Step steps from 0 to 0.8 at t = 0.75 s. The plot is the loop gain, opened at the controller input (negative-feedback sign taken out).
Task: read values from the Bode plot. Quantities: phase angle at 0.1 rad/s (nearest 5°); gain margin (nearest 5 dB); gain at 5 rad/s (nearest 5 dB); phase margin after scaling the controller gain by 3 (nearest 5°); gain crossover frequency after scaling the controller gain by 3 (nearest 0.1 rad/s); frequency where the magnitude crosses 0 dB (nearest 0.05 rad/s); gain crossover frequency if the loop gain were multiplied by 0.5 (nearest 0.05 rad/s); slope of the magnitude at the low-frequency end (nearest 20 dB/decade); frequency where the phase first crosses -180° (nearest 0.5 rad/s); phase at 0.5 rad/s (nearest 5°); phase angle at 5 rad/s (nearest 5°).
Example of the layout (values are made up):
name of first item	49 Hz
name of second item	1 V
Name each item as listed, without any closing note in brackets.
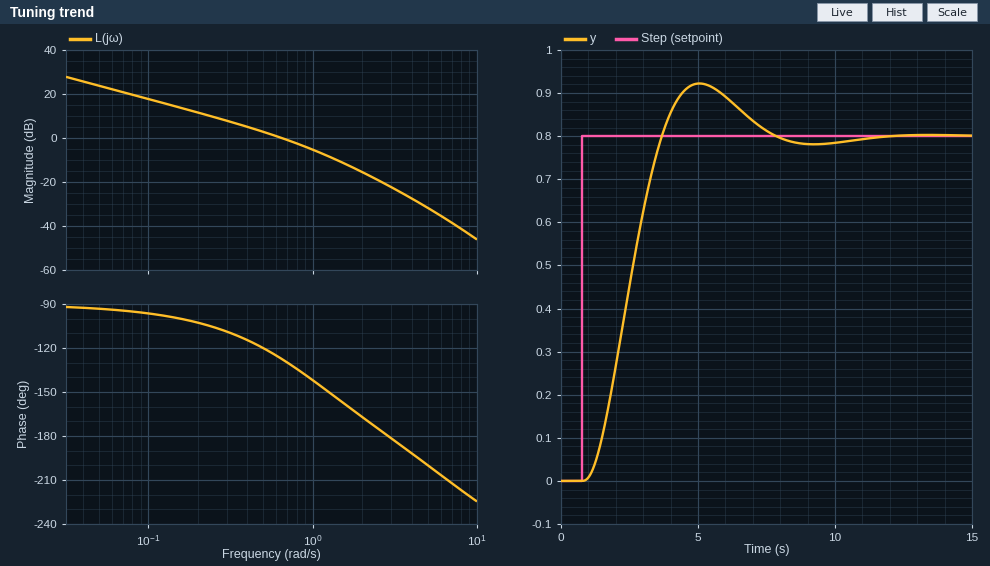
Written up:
phase angle at 0.1 rad/s	-95°
gain margin	20 dB
gain at 5 rad/s	-30 dB
phase margin after scaling the controller gain by 3	25°
gain crossover frequency after scaling the controller gain by 3	1.4 rad/s
frequency where the magnitude crosses 0 dB	0.65 rad/s
gain crossover frequency if the loop gain were multiplied by 0.5	0.35 rad/s
slope of the magnitude at the low-frequency end	-20 dB/decade
frequency where the phase first crosses -180°	3.0 rad/s
phase at 0.5 rad/s	-120°
phase angle at 5 rad/s	-200°
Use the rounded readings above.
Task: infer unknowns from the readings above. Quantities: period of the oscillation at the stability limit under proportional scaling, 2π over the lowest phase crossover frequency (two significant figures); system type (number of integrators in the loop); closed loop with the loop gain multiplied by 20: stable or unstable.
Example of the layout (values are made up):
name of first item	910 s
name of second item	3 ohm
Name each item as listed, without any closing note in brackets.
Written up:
period of the oscillation at the stability limit under proportional scaling, 2π over the lowest phase crossover frequency	2.1 s
system type	1
closed loop with the loop gain multiplied by 20: stable or unstable	unstable
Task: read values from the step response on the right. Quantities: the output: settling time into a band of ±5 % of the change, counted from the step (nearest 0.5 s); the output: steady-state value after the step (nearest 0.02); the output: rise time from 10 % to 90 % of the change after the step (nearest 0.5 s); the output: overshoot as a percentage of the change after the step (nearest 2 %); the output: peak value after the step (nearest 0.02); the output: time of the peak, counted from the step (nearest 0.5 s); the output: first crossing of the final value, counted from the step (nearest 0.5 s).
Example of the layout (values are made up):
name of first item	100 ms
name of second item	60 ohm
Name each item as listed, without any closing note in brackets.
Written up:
the output: settling time into a band of ±5 % of the change, counted from the step	6.0 s
the output: steady-state value after the step	0.80
the output: rise time from 10 % to 90 % of the change after the step	2.0 s
the output: overshoot as a percentage of the change after the step	16 %
the output: peak value after the step	0.92
the output: time of the peak, counted from the step	4.5 s
the output: first crossing of the final value, counted from the step	3.0 s
